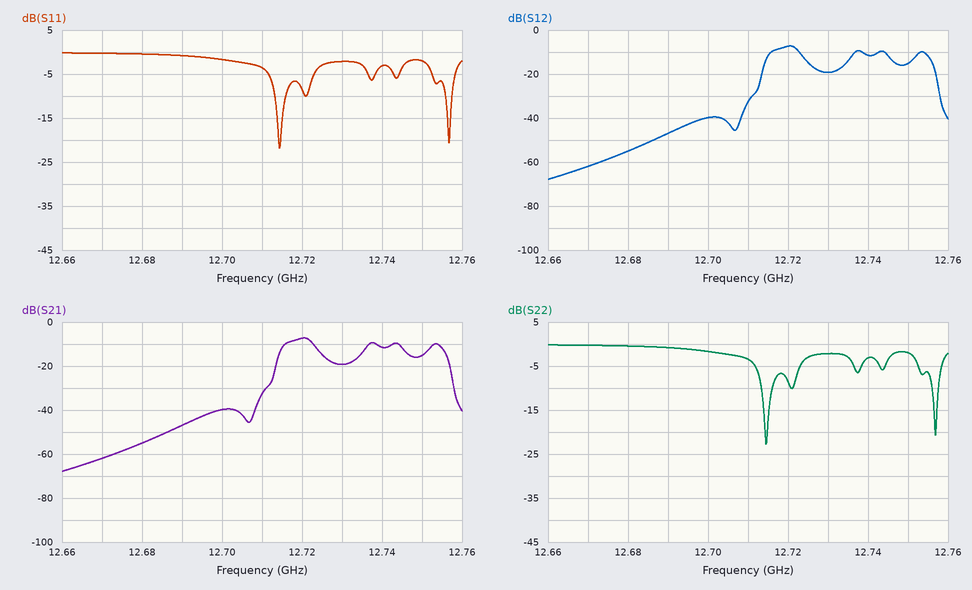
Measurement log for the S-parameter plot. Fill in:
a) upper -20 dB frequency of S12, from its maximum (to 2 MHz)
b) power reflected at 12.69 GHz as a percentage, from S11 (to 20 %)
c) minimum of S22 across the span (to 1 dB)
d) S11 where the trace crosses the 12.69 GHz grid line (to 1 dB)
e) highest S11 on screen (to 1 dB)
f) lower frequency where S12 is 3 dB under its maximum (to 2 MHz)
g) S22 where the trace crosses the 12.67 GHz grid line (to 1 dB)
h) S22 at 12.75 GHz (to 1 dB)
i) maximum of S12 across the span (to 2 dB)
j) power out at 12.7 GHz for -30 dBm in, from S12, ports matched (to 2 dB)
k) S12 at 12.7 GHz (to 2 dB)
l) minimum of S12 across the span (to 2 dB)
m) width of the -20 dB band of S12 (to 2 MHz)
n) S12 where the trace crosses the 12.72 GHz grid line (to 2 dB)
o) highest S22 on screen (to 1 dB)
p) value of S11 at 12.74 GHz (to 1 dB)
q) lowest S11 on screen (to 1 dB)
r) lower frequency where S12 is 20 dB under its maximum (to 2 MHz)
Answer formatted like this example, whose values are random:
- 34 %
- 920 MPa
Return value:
- 12.758 GHz
- 80 %
- -23 dB
- -1 dB
- 0 dB
- 12.716 GHz
- 0 dB
- -2 dB
- -8 dB
- -70 dBm
- -40 dB
- -68 dB
- 46 MHz
- -8 dB
- 0 dB
- -3 dB
- -22 dB
- 12.712 GHz
